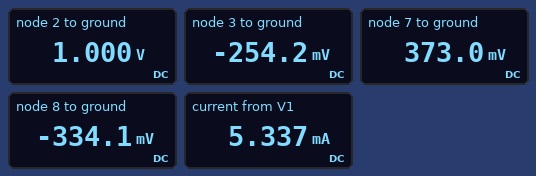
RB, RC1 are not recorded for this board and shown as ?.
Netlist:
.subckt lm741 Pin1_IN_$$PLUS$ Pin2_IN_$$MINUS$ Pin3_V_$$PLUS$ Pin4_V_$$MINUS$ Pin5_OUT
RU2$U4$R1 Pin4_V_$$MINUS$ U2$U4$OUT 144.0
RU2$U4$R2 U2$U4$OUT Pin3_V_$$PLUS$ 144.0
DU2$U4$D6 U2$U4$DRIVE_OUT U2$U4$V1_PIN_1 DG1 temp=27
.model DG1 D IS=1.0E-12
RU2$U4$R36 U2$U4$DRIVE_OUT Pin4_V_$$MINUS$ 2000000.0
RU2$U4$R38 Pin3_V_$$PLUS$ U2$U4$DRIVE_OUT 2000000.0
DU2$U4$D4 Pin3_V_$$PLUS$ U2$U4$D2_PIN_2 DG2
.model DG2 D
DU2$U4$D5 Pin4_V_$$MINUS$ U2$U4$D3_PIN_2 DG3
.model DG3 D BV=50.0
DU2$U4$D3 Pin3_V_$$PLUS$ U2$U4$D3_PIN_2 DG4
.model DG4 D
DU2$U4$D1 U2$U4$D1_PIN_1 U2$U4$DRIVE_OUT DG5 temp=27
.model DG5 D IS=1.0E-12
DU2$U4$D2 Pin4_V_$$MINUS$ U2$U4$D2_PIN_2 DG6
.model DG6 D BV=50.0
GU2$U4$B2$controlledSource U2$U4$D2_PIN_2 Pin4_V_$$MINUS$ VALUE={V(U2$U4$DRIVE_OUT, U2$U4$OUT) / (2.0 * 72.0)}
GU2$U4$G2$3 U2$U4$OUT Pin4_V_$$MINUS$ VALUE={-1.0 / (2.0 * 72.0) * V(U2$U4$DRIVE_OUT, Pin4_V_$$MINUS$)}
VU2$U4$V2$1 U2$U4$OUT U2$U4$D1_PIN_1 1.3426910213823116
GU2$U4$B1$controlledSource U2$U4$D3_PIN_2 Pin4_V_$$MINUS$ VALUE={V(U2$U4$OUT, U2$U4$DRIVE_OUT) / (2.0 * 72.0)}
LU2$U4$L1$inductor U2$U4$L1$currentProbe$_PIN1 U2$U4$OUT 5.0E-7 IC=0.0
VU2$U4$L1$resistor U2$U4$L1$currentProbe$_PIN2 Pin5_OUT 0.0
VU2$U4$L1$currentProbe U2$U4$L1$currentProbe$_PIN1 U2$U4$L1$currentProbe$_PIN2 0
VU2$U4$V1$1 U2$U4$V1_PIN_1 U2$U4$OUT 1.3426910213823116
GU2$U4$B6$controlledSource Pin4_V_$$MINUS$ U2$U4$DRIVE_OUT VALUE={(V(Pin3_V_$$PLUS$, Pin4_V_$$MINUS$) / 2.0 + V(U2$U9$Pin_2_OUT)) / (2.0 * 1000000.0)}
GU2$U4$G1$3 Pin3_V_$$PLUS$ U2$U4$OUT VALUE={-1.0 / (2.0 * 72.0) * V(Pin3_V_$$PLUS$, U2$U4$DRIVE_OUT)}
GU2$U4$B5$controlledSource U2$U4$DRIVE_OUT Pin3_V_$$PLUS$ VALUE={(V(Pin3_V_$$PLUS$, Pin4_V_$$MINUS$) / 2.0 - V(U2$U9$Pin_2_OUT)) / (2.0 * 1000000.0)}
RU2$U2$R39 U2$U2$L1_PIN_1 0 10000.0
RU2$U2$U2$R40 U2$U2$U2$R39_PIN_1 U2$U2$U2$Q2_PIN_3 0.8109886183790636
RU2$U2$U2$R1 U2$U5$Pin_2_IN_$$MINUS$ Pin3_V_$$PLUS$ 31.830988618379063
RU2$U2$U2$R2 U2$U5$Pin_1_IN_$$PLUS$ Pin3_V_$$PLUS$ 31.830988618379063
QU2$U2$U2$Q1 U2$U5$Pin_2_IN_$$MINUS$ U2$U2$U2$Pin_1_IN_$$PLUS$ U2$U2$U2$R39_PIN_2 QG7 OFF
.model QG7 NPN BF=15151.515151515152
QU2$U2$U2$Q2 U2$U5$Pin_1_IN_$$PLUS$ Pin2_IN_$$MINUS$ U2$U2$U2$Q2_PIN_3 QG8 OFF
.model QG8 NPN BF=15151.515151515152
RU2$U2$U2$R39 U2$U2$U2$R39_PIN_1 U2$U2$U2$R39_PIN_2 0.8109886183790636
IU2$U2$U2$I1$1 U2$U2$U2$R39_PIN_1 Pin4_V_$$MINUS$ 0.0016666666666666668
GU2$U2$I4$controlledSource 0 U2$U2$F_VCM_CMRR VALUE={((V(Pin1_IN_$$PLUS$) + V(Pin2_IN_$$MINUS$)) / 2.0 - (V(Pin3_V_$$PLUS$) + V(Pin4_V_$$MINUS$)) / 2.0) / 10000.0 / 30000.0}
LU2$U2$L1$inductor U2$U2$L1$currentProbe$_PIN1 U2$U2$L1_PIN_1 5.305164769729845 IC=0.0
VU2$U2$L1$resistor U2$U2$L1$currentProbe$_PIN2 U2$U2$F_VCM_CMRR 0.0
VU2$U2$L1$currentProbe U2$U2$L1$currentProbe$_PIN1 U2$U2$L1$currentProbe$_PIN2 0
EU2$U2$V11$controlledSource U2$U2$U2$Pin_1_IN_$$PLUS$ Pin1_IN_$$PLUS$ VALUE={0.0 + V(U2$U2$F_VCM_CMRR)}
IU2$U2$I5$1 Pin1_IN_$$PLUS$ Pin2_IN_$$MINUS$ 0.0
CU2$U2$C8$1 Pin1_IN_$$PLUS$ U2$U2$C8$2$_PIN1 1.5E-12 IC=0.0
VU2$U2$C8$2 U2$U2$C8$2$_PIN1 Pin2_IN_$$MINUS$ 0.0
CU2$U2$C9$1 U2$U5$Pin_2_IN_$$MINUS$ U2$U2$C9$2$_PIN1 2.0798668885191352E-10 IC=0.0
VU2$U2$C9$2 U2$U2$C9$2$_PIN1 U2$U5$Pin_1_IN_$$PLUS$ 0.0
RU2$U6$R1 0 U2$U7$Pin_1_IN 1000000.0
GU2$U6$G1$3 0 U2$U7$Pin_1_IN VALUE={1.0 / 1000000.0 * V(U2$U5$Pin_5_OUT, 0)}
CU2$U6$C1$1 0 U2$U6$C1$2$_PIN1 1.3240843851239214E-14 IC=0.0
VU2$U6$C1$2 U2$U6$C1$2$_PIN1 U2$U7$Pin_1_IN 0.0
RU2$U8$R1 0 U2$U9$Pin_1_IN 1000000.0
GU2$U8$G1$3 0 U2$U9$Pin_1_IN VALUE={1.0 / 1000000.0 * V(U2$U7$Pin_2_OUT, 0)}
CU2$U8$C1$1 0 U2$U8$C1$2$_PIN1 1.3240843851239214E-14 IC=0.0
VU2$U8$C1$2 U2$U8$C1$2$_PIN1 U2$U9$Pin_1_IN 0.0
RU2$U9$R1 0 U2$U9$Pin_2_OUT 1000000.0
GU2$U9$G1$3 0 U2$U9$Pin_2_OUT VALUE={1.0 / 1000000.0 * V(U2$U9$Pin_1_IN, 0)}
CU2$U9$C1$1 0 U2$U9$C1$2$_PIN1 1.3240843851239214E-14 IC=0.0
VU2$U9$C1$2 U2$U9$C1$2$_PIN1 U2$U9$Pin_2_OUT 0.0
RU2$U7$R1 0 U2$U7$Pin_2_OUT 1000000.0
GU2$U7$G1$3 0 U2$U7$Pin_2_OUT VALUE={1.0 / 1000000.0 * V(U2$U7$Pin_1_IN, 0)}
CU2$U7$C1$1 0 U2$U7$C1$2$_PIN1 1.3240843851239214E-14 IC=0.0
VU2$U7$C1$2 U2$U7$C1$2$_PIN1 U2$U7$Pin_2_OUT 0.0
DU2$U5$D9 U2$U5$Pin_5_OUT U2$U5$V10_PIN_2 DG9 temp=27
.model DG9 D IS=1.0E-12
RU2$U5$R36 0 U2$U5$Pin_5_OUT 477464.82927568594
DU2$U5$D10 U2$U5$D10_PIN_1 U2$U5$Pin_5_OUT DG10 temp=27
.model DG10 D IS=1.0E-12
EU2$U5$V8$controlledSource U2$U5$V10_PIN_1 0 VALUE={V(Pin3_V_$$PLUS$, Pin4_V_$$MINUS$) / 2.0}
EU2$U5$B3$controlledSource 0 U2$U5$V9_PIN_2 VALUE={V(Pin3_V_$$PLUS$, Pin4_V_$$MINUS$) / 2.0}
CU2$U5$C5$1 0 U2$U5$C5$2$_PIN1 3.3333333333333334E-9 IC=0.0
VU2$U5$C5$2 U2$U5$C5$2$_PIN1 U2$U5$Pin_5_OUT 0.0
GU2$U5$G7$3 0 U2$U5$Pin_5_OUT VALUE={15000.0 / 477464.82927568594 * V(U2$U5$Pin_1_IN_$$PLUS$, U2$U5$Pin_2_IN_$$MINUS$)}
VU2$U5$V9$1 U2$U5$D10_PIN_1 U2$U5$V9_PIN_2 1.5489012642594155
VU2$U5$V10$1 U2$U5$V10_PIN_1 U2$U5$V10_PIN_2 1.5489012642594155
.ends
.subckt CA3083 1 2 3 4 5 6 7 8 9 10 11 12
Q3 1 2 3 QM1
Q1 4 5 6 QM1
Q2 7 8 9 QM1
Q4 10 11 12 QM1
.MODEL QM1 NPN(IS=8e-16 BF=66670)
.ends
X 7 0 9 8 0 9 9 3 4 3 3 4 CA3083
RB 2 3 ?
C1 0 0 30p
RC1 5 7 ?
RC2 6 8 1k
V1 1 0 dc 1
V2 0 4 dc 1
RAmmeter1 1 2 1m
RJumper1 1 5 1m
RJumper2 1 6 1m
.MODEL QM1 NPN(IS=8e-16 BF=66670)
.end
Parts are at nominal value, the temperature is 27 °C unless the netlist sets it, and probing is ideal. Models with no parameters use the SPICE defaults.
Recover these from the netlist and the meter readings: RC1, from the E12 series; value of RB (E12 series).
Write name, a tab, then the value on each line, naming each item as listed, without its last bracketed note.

RC1, from the E12 series	470 Ω
value of RB	470 Ω
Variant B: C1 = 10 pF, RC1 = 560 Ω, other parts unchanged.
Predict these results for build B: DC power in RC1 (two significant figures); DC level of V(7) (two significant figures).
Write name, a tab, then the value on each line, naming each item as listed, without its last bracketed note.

DC power in RC1	1.0 mW
DC level of V(7)	250 mV
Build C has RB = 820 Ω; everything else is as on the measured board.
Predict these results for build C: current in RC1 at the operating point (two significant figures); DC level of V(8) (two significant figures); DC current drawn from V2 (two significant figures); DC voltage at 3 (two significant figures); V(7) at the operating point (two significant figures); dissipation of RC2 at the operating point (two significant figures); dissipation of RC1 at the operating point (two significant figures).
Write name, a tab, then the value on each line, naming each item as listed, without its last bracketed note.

current in RC1 at the operating point	770 µA
DC level of V(8)	230 mV
DC current drawn from V2	3.1 mA
DC voltage at 3	-270 mV
V(7) at the operating point	640 mV
dissipation of RC2 at the operating point	600 µW
dissipation of RC1 at the operating point	280 µW
